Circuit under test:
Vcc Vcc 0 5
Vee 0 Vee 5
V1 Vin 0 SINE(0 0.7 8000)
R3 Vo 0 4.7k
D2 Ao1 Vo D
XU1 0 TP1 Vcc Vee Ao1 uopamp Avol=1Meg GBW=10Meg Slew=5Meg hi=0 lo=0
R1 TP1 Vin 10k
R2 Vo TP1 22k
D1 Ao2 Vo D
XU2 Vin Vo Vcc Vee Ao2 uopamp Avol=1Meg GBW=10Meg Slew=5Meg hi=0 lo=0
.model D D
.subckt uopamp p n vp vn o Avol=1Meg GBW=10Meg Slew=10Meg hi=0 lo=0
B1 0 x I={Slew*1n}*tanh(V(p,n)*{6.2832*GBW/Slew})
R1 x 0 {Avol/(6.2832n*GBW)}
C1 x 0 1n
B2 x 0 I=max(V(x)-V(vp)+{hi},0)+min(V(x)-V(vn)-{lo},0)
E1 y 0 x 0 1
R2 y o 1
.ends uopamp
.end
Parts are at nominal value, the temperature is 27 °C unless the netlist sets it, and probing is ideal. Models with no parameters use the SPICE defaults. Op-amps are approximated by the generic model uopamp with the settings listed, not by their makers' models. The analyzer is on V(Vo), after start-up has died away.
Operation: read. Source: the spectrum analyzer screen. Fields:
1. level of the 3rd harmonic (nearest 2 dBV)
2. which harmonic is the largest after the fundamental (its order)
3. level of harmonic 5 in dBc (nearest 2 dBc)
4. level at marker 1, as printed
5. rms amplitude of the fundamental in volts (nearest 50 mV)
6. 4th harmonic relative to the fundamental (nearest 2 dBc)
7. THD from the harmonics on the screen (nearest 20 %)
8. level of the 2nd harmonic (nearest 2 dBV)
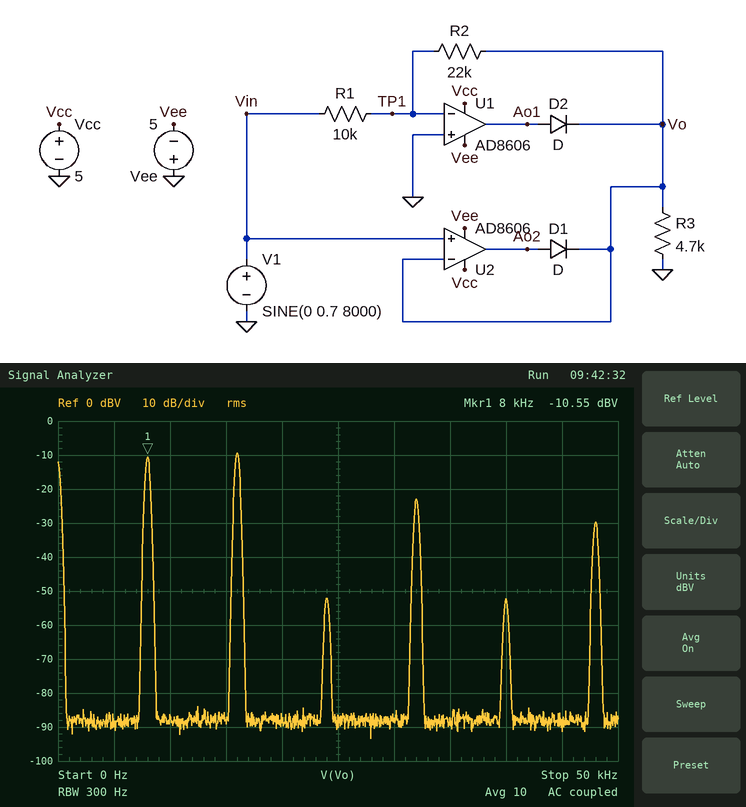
-52 dBV
2
-42 dBc
-10.55 dBV
300 mV
-12 dBc
120 %
-10 dBV
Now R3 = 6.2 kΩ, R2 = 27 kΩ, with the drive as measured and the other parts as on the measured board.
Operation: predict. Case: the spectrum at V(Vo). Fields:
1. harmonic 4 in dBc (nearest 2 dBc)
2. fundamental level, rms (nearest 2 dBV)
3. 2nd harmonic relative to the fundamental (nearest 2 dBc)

-14 dBc
-8 dBV
0 dBc
